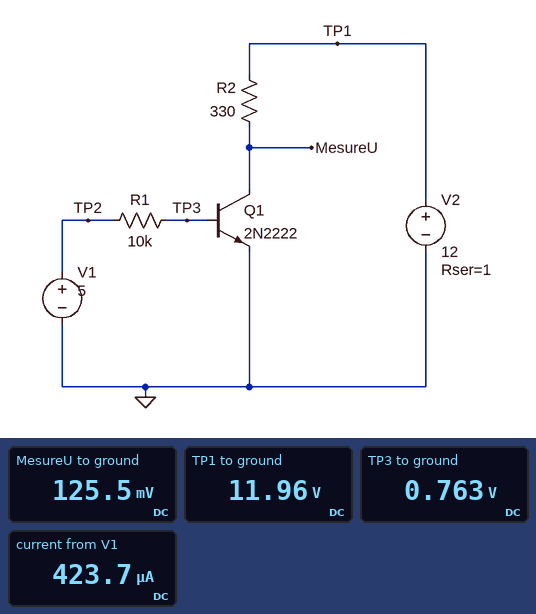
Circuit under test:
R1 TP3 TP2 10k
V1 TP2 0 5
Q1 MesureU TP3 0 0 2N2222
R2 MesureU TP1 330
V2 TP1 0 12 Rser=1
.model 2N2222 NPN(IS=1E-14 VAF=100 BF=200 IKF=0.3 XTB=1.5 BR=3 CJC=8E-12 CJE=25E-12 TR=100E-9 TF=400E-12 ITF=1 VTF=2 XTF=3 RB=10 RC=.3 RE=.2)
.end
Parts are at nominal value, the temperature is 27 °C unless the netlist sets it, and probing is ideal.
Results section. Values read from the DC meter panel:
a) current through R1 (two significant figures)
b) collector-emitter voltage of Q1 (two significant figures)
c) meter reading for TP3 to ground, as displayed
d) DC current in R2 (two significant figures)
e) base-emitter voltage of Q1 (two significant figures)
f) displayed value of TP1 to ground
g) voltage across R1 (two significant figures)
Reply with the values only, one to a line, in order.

420 µA
130 mV
0.763 V
36 mA
760 mV
11.96 V
4.2 V
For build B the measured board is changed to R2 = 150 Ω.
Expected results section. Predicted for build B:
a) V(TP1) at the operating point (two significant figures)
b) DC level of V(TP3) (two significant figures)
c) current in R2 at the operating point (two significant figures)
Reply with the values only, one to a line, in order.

12 V
790 mV
69 mA
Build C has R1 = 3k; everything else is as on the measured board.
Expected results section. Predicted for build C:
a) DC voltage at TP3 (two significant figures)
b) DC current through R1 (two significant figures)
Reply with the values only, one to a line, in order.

780 mV
1.4 mA
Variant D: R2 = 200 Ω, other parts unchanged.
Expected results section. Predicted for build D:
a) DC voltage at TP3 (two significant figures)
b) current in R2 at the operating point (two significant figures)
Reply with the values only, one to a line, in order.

780 mV
59 mA
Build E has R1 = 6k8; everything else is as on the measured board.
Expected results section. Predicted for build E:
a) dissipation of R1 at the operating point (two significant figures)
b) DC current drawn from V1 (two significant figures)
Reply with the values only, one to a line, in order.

2.6 mW
620 µA
